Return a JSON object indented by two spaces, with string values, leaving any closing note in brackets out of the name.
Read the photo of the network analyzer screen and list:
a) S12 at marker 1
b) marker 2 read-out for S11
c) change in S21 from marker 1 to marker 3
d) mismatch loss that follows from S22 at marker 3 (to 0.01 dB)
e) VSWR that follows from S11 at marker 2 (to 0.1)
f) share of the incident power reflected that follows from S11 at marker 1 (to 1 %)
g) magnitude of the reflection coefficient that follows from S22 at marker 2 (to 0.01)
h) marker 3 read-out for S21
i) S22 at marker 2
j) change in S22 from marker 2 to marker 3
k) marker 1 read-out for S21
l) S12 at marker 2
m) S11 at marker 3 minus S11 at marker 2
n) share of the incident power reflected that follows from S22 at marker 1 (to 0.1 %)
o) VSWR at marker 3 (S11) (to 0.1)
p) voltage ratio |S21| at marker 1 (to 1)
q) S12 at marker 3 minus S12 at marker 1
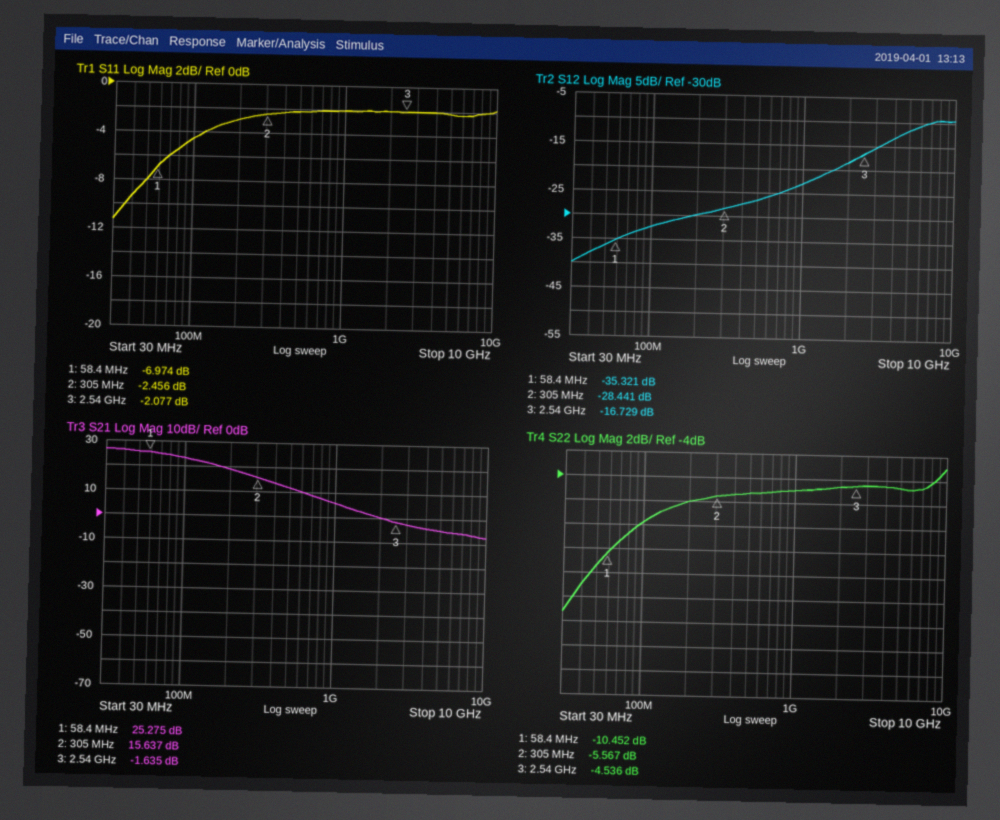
{
  "S12 at marker 1": "-35.321 dB",
  "marker 2 read-out for S11": "-2.456 dB",
  "change in S21 from marker 1 to marker 3": "-26.910 dB",
  "mismatch loss that follows from S22 at marker 3": "1.88 dB",
  "VSWR that follows from S11 at marker 2": "7.1",
  "share of the incident power reflected that follows from S11 at marker 1": "20 %",
  "magnitude of the reflection coefficient that follows from S22 at marker 2": "0.53",
  "marker 3 read-out for S21": "-1.635 dB",
  "S22 at marker 2": "-5.567 dB",
  "change in S22 from marker 2 to marker 3": "1.031 dB",
  "marker 1 read-out for S21": "25.275 dB",
  "S12 at marker 2": "-28.441 dB",
  "S11 at marker 3 minus S11 at marker 2": "0.379 dB",
  "share of the incident power reflected that follows from S22 at marker 1": "9.0 %",
  "VSWR at marker 3 (S11)": "8.4",
  "voltage ratio |S21| at marker 1": "18",
  "S12 at marker 3 minus S12 at marker 1": "18.592 dB"
}
